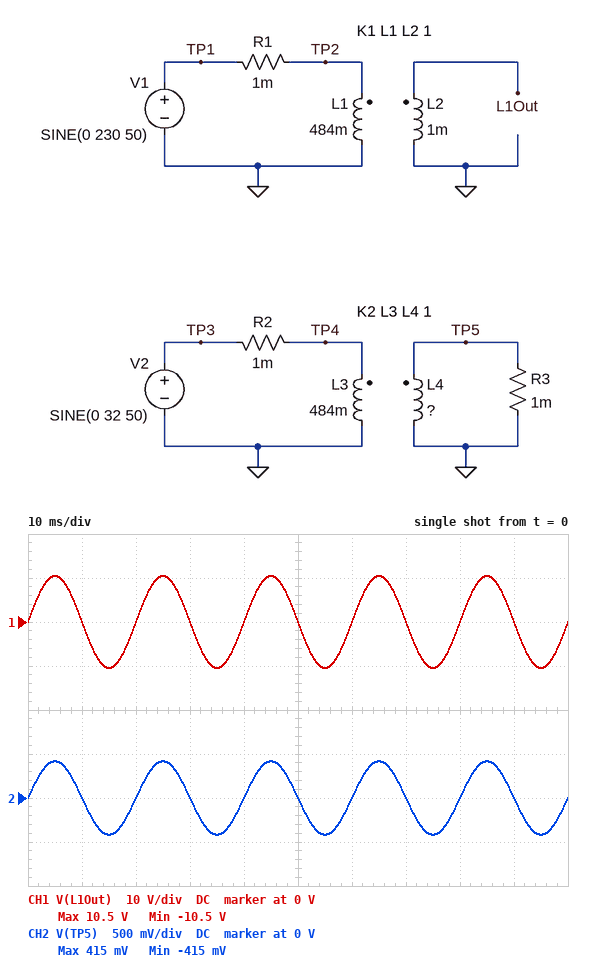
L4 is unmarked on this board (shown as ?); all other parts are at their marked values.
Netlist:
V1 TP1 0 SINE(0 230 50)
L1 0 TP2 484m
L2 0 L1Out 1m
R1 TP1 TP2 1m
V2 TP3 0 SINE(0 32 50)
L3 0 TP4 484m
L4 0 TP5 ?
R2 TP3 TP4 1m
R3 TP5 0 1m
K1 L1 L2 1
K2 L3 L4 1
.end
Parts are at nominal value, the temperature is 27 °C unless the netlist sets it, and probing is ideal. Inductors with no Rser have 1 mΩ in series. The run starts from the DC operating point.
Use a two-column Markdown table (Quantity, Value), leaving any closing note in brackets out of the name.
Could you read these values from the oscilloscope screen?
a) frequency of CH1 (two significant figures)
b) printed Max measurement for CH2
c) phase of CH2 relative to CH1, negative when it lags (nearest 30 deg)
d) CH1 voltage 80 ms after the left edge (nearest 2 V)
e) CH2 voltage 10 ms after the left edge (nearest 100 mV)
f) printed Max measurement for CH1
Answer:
| Quantity | Value |
|---|---|
| frequency of CH1 | 50 Hz |
| printed Max measurement for CH2 | 415 mV |
| phase of CH2 relative to CH1, negative when it lags | 0 deg |
| CH1 voltage 80 ms after the left edge | 0 V |
| CH2 voltage 10 ms after the left edge | 0 V |
| printed Max measurement for CH1 | 10.5 V |
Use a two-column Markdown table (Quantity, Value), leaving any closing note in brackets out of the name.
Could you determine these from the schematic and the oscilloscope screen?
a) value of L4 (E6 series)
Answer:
| Quantity | Value |
|---|---|
| value of L4 | 330 µH |
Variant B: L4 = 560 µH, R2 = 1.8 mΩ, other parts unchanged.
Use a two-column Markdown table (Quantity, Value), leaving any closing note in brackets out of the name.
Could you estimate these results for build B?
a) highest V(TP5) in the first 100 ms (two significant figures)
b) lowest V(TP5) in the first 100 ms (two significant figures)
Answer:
| Quantity | Value |
|---|---|
| highest V(TP5) in the first 100 ms | 540 mV |
| lowest V(TP5) in the first 100 ms | -540 mV |
